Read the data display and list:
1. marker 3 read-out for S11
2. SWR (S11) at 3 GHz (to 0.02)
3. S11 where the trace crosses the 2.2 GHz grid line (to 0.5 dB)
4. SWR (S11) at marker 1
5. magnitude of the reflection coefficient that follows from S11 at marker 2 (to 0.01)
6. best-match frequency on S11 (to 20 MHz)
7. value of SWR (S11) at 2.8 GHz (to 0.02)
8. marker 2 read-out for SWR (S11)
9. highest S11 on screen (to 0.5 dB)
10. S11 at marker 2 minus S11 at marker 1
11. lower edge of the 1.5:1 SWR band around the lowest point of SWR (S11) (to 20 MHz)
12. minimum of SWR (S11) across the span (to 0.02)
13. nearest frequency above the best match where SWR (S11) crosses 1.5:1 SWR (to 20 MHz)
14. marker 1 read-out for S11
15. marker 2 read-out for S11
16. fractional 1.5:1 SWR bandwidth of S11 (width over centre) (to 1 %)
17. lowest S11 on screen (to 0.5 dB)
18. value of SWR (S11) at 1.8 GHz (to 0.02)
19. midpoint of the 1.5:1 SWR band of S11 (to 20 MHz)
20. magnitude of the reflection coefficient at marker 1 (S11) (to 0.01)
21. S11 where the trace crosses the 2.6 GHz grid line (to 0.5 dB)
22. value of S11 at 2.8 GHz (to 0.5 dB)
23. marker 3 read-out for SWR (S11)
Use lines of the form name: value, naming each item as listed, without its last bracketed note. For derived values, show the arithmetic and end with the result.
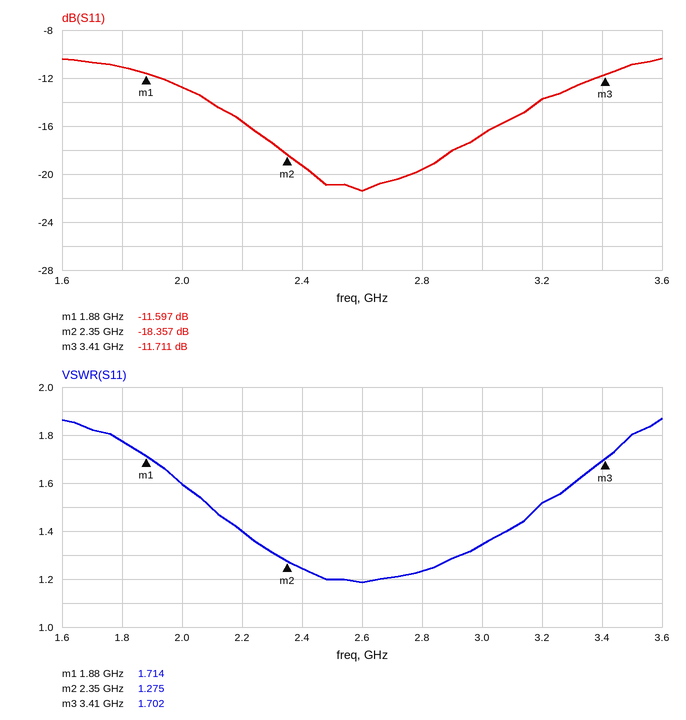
marker 3 read-out for S11: -11.711 dB
SWR (S11) at 3 GHz: 1.34
S11 where the trace crosses the 2.2 GHz grid line: -15.5 dB
SWR (S11) at marker 1: 1.714
magnitude of the reflection coefficient that follows from S11 at marker 2: 10^(-18.357/20) ≈ 0.12
best-match frequency on S11: 2.60 GHz
value of SWR (S11) at 2.8 GHz: 1.24
marker 2 read-out for SWR: 1.275
highest S11 on screen: -10.5 dB
S11 at marker 2 minus S11 at marker 1: -18.357 − (-11.597) = -6.760 dB
lower edge of the 1.5:1 SWR band around the lowest point of SWR (S11): 2.10 GHz
minimum of SWR (S11) across the span: 1.18
nearest frequency above the best match where SWR (S11) crosses 1.5:1 SWR: 3.18 GHz
marker 1 read-out for S11: -11.597 dB
marker 2 read-out for S11: -18.357 dB
fractional 1.5:1 SWR bandwidth of S11 (width over centre): 1.08 GHz / 2.64 GHz ≈ 41 %
lowest S11 on screen: -21.5 dB
value of SWR (S11) at 1.8 GHz: 1.78
midpoint of the 1.5:1 SWR band of S11: 2.64 GHz
magnitude of the reflection coefficient at marker 1 (S11): 10^(-11.597/20) ≈ 0.26
S11 where the trace crosses the 2.6 GHz grid line: -21.5 dB
value of S11 at 2.8 GHz: -19.5 dB
marker 3 read-out for SWR: 1.702
